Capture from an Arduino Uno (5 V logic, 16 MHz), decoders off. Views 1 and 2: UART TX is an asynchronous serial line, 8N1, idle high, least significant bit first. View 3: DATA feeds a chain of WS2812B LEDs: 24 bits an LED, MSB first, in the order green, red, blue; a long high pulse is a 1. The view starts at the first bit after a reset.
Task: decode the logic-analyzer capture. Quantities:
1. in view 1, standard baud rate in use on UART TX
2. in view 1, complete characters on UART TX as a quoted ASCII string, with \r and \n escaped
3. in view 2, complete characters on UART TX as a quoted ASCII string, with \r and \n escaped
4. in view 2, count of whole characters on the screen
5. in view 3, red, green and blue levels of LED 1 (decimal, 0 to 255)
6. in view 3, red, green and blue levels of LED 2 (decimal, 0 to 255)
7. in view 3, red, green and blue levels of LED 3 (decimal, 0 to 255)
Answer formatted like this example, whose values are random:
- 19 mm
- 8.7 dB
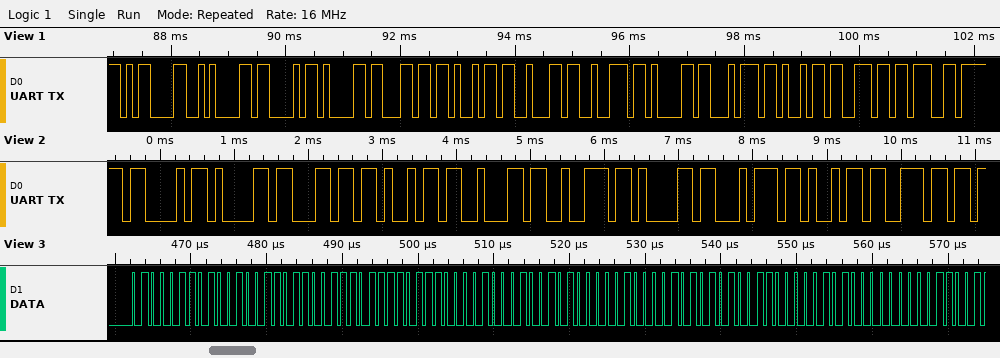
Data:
- 9600 baud
- "\r\nCalibrating"
- "Calibratin"
- 10
- 147, 70, 103
- 132, 123, 74
- 85, 8, 48
